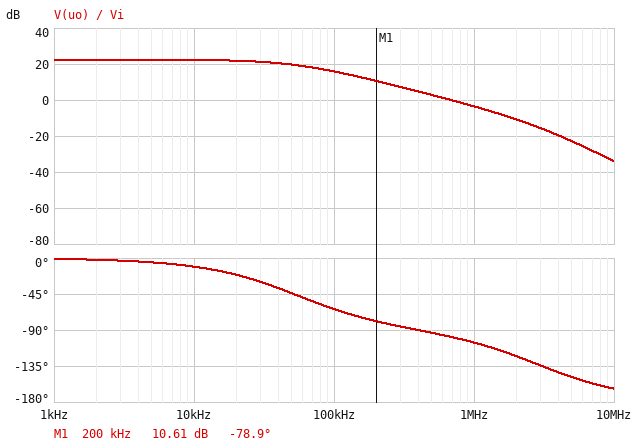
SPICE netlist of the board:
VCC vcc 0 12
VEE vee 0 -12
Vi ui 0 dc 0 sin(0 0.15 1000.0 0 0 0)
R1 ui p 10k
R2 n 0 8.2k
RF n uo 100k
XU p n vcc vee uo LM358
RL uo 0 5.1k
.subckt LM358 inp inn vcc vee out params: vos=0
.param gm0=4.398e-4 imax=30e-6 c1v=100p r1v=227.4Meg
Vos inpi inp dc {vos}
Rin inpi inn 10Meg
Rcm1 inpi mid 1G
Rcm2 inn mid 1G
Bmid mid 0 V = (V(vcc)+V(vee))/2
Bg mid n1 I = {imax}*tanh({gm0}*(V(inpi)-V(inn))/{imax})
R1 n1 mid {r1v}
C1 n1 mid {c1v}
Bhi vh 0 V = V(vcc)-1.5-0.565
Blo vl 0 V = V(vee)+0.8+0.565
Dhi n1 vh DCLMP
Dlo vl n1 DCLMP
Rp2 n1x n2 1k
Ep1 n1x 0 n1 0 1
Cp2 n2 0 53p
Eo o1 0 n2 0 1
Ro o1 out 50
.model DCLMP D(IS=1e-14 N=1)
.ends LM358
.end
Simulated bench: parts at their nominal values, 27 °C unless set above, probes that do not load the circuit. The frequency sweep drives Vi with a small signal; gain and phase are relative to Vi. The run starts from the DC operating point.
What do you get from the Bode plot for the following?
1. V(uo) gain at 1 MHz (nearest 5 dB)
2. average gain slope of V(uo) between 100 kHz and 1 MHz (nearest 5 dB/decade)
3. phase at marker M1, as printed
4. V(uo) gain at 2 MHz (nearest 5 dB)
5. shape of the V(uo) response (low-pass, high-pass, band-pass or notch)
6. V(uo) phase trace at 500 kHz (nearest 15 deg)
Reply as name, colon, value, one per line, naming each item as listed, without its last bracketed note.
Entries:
V(uo) gain at 1 MHz: -5 dB
average gain slope of V(uo) between 100 kHz and 1 MHz: -20 dB/decade
phase at marker M1, as printed: -78.9 deg
V(uo) gain at 2 MHz: -10 dB
shape of the V(uo) response: low-pass
V(uo) phase trace at 500 kHz: -90 deg
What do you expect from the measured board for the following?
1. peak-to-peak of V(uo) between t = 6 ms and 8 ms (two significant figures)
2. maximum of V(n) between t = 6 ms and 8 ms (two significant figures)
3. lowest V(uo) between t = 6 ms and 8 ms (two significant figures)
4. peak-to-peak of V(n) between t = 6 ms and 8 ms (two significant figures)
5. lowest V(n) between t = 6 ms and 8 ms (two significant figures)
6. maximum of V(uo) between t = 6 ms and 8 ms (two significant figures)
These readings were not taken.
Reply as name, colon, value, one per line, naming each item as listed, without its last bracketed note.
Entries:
peak-to-peak of V(uo) between t = 6 ms and 8 ms: 4.0 V
maximum of V(n) between t = 6 ms and 8 ms: 150 mV
lowest V(uo) between t = 6 ms and 8 ms: -2.0 V
peak-to-peak of V(n) between t = 6 ms and 8 ms: 300 mV
lowest V(n) between t = 6 ms and 8 ms: -150 mV
maximum of V(uo) between t = 6 ms and 8 ms: 2.0 V
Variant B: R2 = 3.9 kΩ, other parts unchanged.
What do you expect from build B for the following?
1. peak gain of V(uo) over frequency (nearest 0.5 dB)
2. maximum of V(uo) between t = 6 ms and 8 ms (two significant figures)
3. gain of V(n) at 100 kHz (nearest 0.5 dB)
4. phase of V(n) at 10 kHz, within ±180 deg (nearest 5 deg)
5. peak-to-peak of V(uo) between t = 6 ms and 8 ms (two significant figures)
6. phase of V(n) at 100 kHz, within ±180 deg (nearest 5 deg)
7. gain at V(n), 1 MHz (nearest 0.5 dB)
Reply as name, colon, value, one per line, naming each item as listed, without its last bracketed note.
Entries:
peak gain of V(uo) over frequency: 28.5 dB
maximum of V(uo) between t = 6 ms and 8 ms: 4.0 V
gain of V(n) at 100 kHz: -12.0 dB
phase of V(n) at 10 kHz, within ±180 deg: -20 deg
peak-to-peak of V(uo) between t = 6 ms and 8 ms: 8.0 V
phase of V(n) at 100 kHz, within ±180 deg: -75 deg
gain at V(n), 1 MHz: -32.0 dB
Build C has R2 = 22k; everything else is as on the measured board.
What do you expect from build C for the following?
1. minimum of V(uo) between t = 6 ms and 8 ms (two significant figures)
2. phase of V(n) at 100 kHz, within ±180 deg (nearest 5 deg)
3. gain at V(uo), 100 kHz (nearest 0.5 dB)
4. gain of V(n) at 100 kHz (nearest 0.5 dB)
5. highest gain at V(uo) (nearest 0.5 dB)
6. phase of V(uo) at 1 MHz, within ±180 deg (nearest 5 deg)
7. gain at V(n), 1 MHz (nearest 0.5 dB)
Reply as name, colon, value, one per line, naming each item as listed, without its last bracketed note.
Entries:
minimum of V(uo) between t = 6 ms and 8 ms: -830 mV
phase of V(n) at 100 kHz, within ±180 deg: -40 deg
gain at V(uo), 100 kHz: 13.0 dB
gain of V(n) at 100 kHz: -2.0 dB
highest gain at V(uo): 15.0 dB
phase of V(uo) at 1 MHz, within ±180 deg: -100 deg
gain at V(n), 1 MHz: -18.5 dB
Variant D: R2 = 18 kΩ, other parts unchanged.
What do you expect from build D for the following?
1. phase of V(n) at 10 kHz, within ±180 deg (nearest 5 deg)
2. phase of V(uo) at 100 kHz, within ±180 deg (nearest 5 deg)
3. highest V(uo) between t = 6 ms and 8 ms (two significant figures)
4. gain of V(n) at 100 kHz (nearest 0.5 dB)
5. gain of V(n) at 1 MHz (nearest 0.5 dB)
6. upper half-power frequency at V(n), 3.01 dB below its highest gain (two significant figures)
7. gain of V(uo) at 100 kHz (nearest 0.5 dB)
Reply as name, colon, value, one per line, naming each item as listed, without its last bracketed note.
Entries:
phase of V(n) at 10 kHz, within ±180 deg: -5 deg
phase of V(uo) at 100 kHz, within ±180 deg: -45 deg
highest V(uo) between t = 6 ms and 8 ms: 980 mV
gain of V(n) at 100 kHz: -2.5 dB
gain of V(n) at 1 MHz: -20.0 dB
upper half-power frequency at V(n), 3.01 dB below its highest gain: 110 kHz
gain of V(uo) at 100 kHz: 13.5 dB
